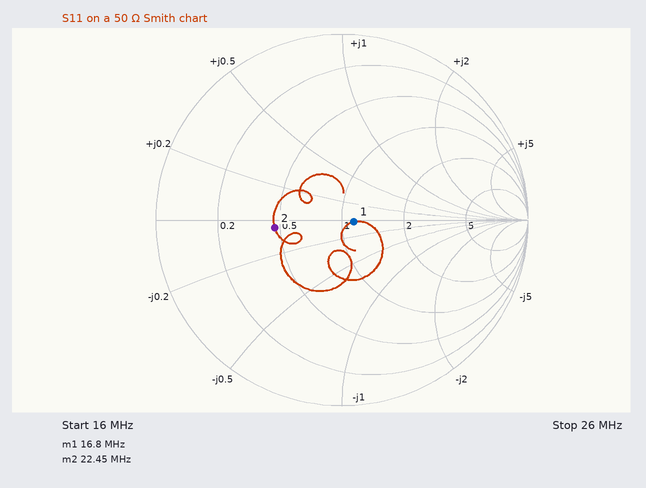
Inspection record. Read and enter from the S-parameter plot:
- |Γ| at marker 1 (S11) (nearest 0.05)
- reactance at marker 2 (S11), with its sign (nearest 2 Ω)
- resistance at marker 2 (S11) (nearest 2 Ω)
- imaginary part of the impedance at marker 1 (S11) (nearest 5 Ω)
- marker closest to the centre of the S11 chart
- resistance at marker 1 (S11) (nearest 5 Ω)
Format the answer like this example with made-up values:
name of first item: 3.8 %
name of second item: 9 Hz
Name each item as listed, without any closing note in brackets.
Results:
|Γ| at marker 1 (S11): 0.05
reactance at marker 2 (S11), with its sign: -2 Ω
resistance at marker 2 (S11): 24 Ω
imaginary part of the impedance at marker 1 (S11): 0 Ω
marker closest to the centre of the S11 chart: marker 1
resistance at marker 1 (S11): 55 Ω
